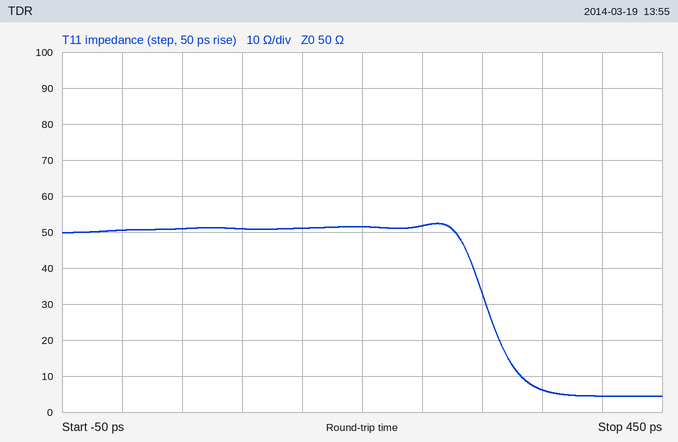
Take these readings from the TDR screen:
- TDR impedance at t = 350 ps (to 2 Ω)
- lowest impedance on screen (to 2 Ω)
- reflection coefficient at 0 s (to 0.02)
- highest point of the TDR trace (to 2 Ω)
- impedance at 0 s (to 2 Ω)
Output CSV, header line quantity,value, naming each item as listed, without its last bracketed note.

quantity,value
TDR impedance at t = 350 ps,6 Ω
lowest impedance on screen,4 Ω
reflection coefficient at 0 s,0.00
highest point of the TDR trace,52 Ω
impedance at 0 s,50 Ω
